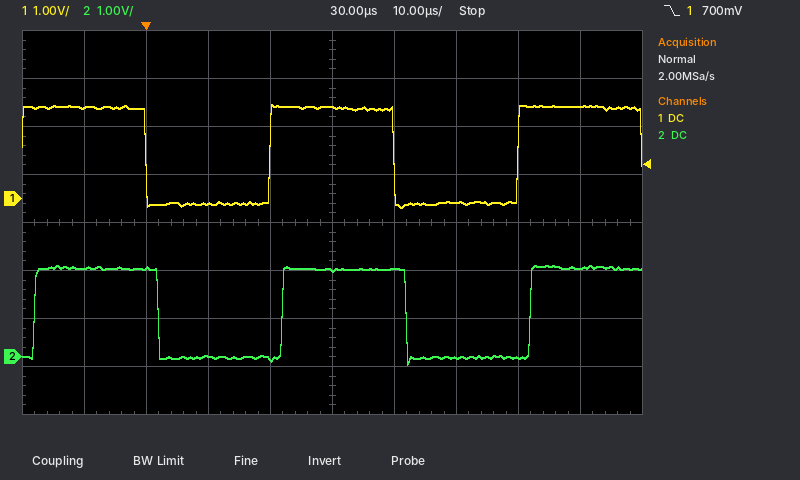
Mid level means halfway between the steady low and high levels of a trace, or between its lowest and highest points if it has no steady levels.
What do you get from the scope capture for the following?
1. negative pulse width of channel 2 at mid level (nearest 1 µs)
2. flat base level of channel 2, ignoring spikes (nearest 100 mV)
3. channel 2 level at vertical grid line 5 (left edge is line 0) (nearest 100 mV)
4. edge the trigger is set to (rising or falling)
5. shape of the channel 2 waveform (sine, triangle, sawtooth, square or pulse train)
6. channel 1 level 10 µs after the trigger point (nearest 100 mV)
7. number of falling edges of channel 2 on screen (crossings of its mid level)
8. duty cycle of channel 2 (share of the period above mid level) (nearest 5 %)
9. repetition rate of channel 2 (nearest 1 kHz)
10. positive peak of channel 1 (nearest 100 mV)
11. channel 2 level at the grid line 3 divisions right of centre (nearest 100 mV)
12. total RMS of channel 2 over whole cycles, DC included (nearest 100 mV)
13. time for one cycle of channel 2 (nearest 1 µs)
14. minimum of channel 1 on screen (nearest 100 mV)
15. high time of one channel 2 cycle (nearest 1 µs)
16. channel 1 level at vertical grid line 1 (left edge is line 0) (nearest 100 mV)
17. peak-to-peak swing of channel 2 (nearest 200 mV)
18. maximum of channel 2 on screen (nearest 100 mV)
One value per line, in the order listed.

20 µs
0.0 V
1.8 V
falling
square
-100 mV
2
50 %
25 kHz
2.0 V
0.0 V
1.3 V
40 µs
-200 mV
20 µs
1.9 V
2.0 V
1.9 V
